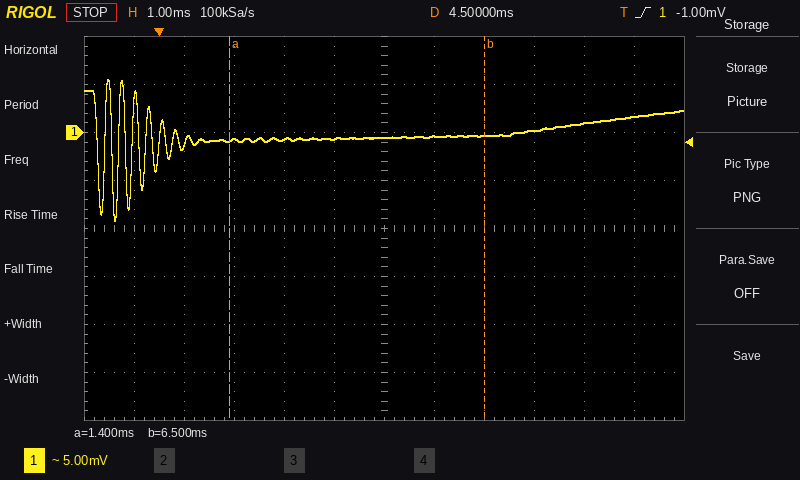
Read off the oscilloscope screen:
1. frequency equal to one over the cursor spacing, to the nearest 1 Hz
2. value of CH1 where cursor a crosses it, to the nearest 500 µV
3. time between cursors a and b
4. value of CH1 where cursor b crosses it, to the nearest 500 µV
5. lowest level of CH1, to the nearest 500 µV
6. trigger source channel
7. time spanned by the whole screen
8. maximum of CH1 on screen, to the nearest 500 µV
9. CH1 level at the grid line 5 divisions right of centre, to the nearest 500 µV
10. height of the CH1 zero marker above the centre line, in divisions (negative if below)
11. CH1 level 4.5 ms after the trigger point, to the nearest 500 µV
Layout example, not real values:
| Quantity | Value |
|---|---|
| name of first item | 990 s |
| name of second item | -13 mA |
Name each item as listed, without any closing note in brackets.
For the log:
| Quantity | Value |
|---|---|
| frequency equal to one over the cursor spacing, to the nearest 1 Hz | 196 Hz |
| value of CH1 where cursor a crosses it, to the nearest 500 µV | -1.0 mV |
| time between cursors a and b | 5.1 ms |
| value of CH1 where cursor b crosses it, to the nearest 500 µV | -500 µV |
| lowest level of CH1, to the nearest 500 µV | -9.0 mV |
| trigger source channel | CH1 |
| time spanned by the whole screen | 12 ms |
| maximum of CH1 on screen, to the nearest 500 µV | 5.5 mV |
| CH1 level at the grid line 5 divisions right of centre, to the nearest 500 µV | 1.5 mV |
| height of the CH1 zero marker above the centre line, in divisions | +2.0 div |
| CH1 level 4.5 ms after the trigger point, to the nearest 500 µV | -500 µV |
